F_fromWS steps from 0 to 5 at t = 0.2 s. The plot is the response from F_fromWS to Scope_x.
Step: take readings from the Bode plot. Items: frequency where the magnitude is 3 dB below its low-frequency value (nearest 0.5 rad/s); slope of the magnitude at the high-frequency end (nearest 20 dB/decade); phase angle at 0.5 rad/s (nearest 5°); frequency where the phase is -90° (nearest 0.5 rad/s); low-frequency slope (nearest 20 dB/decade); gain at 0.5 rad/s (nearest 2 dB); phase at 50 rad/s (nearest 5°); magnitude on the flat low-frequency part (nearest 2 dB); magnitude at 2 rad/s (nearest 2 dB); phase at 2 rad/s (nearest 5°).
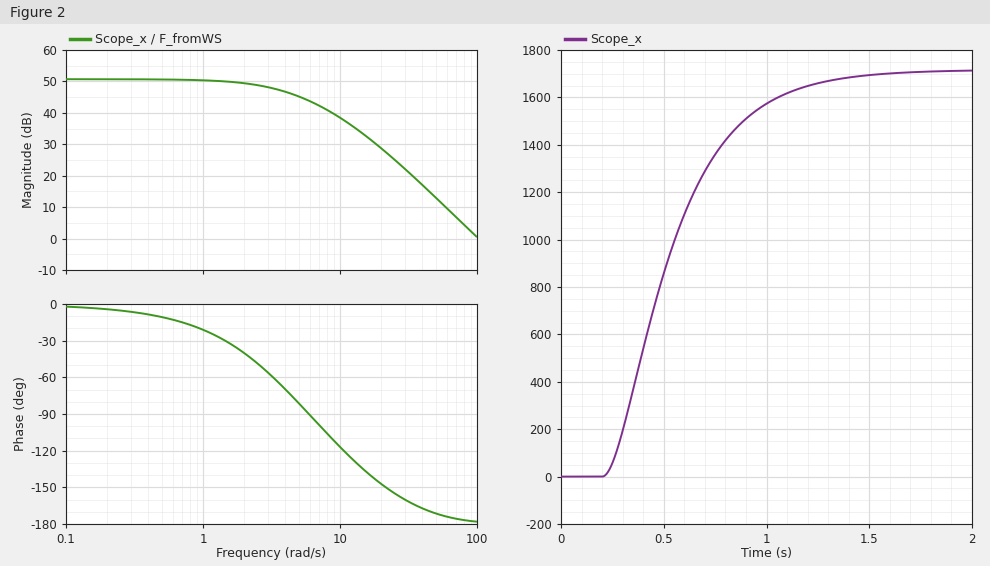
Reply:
3.5 rad/s
-40 dB/decade
-10°
6.0 rad/s
0 dB/decade
50 dB
-170°
50 dB
50 dB
-40°
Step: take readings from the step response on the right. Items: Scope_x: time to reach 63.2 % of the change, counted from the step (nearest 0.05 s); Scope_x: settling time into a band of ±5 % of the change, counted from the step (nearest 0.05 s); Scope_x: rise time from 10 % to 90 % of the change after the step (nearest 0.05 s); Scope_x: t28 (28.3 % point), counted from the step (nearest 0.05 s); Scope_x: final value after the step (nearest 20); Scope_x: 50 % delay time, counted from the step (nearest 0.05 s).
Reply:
0.40 s
0.95 s
0.65 s
0.20 s
1720
0.30 s
